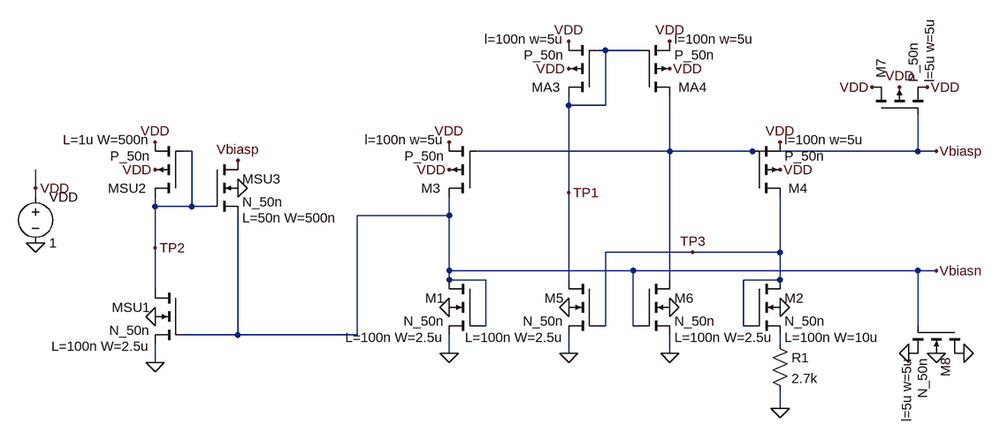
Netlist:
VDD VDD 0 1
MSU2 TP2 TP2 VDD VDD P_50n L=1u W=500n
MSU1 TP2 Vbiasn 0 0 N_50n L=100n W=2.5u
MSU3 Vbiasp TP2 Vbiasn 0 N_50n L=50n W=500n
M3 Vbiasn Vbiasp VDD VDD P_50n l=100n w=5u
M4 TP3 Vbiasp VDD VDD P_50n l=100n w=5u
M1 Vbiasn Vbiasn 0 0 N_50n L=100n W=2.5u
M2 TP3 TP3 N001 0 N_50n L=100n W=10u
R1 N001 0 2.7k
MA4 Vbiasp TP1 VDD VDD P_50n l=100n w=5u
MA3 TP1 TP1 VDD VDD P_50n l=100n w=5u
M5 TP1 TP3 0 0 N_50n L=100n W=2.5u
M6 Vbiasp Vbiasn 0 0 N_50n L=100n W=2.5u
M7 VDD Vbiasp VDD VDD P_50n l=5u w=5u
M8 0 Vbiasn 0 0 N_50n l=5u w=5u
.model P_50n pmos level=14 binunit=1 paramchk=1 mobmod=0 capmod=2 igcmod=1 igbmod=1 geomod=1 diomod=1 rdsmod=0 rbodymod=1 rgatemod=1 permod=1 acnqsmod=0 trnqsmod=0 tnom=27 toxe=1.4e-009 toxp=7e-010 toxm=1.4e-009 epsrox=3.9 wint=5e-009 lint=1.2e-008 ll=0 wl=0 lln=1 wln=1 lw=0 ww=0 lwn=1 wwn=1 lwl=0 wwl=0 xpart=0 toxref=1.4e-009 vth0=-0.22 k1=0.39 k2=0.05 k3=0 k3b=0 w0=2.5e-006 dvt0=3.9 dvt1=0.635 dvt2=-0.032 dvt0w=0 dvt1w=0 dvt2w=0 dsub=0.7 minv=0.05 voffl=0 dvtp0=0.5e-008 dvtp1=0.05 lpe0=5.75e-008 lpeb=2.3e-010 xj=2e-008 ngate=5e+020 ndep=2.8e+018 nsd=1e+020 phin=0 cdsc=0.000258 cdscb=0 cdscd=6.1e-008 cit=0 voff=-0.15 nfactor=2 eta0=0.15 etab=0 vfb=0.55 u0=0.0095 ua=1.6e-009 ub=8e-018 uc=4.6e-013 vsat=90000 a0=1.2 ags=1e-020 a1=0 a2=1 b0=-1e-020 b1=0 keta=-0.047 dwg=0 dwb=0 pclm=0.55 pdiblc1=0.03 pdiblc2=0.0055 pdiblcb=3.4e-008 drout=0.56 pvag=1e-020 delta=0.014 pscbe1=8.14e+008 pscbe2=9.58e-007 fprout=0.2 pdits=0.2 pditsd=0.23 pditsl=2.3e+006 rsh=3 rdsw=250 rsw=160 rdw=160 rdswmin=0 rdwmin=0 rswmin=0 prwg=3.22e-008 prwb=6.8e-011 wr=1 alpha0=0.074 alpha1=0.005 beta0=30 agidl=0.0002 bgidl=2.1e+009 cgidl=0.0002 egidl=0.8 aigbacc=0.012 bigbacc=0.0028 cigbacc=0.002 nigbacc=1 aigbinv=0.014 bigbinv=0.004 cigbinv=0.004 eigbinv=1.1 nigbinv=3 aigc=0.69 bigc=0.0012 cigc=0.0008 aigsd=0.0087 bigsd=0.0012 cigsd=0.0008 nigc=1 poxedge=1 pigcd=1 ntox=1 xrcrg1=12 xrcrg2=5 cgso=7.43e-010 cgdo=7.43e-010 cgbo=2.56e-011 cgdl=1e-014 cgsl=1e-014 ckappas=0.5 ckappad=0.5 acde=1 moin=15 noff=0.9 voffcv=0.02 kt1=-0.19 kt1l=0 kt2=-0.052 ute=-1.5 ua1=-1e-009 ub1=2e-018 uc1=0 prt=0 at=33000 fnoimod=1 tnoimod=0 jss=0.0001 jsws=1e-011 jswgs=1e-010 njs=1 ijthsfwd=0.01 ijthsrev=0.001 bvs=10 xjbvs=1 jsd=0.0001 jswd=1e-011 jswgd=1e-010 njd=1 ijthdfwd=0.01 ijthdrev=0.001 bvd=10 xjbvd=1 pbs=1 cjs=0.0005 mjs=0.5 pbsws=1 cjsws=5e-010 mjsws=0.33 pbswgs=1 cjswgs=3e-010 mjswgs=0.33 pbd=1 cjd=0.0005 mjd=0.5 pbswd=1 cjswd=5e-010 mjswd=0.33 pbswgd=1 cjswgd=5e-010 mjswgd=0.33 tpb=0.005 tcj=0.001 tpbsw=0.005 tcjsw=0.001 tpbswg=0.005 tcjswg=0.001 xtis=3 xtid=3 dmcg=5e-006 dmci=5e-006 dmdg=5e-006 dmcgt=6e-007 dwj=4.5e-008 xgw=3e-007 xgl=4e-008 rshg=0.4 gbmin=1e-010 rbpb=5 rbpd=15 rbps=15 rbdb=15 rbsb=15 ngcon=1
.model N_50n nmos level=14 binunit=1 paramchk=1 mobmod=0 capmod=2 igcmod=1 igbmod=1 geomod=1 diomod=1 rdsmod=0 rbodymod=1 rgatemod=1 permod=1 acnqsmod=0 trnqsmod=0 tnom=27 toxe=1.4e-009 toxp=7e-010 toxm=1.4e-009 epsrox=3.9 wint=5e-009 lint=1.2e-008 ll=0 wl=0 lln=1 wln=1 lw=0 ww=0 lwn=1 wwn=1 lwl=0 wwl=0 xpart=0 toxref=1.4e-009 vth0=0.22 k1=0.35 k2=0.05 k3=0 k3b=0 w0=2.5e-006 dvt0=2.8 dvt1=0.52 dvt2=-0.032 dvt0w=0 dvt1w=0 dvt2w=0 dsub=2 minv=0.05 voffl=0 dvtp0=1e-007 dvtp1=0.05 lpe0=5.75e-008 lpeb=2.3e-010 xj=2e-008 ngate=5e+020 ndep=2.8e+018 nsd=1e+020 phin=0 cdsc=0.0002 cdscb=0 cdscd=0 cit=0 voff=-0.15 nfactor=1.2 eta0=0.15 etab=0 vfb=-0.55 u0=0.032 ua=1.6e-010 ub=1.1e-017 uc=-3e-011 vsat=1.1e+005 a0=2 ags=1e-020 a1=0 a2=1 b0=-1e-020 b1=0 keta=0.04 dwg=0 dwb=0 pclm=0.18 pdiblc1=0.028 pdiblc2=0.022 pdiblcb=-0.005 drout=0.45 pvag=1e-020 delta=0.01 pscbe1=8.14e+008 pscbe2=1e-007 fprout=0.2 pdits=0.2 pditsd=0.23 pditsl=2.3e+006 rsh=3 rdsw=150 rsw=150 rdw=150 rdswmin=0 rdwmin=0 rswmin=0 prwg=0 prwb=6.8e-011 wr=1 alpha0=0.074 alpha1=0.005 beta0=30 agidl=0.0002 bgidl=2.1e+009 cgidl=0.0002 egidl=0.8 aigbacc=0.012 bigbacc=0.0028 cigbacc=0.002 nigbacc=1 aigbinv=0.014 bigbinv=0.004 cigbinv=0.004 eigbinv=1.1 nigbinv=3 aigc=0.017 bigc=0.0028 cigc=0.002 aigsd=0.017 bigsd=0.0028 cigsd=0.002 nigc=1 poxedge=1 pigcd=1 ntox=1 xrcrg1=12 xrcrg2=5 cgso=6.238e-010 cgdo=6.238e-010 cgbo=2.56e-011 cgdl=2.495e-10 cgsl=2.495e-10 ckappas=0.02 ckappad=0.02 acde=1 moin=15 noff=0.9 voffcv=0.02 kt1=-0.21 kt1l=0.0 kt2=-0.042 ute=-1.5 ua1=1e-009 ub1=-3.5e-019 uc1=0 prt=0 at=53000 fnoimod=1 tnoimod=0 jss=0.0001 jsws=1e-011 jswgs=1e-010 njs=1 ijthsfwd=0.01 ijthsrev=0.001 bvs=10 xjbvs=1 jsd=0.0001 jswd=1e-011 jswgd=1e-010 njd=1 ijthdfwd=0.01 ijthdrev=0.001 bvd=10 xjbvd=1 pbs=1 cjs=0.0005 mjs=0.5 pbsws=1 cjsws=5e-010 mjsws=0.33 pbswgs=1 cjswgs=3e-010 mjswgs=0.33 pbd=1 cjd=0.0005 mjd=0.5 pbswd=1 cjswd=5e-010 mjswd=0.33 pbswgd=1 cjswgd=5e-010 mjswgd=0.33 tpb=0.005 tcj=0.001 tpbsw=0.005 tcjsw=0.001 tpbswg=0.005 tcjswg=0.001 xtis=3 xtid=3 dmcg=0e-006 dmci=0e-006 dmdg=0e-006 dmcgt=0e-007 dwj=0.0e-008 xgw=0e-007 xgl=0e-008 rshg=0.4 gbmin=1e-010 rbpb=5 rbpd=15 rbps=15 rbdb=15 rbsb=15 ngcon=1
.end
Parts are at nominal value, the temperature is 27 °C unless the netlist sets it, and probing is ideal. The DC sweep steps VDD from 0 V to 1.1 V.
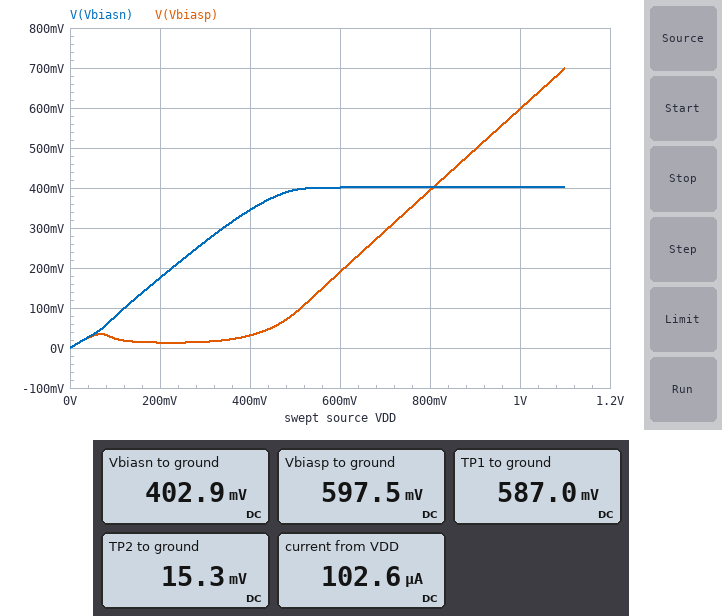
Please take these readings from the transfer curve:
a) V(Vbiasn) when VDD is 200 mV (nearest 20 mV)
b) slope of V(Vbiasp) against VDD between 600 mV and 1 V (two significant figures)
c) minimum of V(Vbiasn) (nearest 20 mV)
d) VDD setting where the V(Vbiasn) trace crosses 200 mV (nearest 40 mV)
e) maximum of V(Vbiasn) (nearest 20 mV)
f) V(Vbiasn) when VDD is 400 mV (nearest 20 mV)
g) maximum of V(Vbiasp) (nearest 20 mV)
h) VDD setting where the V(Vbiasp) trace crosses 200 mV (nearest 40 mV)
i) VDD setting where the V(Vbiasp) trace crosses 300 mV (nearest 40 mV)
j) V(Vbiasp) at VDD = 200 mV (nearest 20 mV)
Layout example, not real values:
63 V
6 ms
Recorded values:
180 mV
1.0 V/V
0 V
240 mV
400 mV
340 mV
700 mV
600 mV
720 mV
20 mV
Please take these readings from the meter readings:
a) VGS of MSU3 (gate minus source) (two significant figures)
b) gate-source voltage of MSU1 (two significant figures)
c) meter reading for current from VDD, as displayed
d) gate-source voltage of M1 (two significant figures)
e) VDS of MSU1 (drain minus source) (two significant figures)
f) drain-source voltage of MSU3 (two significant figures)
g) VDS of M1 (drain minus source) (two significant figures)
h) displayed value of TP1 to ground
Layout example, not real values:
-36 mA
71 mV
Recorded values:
-390 mV
400 mV
102.6 µA
400 mV
15 mV
190 mV
400 mV
587.0 mV
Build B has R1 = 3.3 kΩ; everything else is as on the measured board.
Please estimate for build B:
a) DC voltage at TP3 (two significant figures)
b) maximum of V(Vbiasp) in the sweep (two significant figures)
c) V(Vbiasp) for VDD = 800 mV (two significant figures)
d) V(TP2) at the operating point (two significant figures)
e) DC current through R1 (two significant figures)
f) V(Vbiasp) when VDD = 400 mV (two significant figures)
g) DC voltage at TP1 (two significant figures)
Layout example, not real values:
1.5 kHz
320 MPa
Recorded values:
390 mV
720 mV
410 mV
19 mV
18 µA
35 mV
600 mV
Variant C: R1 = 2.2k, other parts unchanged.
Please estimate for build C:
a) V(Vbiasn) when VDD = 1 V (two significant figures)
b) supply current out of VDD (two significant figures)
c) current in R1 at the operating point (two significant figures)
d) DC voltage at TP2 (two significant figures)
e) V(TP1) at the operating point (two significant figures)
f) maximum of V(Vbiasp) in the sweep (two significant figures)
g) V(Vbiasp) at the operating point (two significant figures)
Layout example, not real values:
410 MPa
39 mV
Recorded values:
420 mV
130 µA
30 µA
13 mV
570 mV
680 mV
580 mV
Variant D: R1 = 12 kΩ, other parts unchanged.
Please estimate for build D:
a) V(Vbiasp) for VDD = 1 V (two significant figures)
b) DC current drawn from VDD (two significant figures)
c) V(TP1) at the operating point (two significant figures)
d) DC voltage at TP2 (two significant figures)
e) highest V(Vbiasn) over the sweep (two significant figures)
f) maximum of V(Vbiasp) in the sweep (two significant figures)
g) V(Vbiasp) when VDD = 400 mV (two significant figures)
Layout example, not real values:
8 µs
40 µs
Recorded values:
700 mV
23 µA
680 mV
210 mV
310 mV
800 mV
89 mV
